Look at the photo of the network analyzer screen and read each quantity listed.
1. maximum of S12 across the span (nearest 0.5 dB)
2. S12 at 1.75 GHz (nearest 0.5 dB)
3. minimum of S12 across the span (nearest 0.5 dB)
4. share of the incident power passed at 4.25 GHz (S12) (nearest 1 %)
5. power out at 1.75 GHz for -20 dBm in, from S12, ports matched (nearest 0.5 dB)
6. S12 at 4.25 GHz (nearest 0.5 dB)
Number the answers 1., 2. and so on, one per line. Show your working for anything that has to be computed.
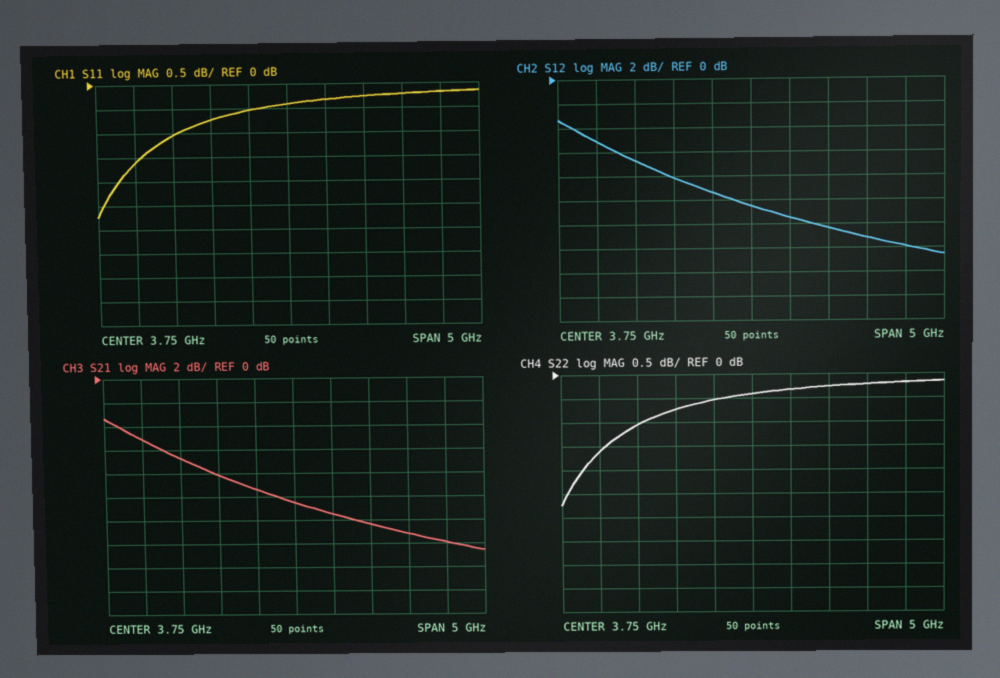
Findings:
1. -3.5 dB
2. -5.0 dB
3. -14.5 dB
4. 10^(-11.5/10) ≈ 7 %
5. -20 dBm + (-5.0 dB) = -25.0 dBm
6. -11.5 dB
